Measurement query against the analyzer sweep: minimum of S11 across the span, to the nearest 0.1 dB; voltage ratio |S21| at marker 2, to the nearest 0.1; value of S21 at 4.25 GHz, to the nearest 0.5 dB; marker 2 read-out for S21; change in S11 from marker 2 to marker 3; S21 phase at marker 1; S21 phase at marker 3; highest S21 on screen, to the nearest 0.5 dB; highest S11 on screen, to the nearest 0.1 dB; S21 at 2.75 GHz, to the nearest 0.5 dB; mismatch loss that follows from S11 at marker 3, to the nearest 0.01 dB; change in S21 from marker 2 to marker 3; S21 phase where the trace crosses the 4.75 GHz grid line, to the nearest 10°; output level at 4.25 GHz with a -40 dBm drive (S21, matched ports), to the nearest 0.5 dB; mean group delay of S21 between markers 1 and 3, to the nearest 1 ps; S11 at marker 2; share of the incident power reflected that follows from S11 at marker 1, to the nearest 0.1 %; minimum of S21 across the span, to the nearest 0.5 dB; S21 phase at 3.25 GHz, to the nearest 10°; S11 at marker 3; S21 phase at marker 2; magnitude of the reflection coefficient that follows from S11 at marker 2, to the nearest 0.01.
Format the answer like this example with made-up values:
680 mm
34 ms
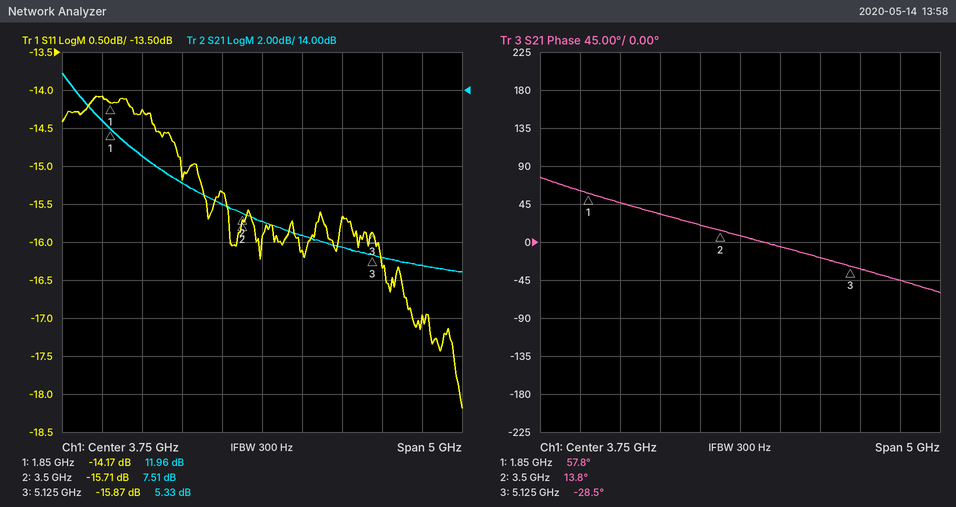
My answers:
-18.2 dB
2.4
6.5 dB
7.51 dB
-0.16 dB
57.8°
-28.5°
15.0 dB
-14.1 dB
9.0 dB
0.11 dB
-2.18 dB
-20°
-33.5 dBm
73 ps
-15.71 dB
3.8 %
4.5 dB
20°
-15.87 dB
13.8°
0.16
